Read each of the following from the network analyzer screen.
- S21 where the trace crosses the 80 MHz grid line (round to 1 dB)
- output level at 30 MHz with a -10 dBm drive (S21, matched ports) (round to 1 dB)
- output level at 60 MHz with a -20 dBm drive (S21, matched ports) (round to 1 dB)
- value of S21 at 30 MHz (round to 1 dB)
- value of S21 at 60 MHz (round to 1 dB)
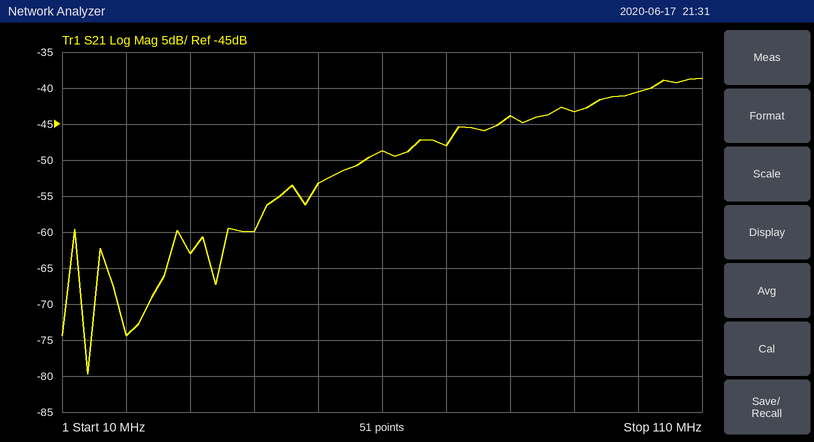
-44 dB
-73 dBm
-69 dBm
-63 dB
-49 dB
